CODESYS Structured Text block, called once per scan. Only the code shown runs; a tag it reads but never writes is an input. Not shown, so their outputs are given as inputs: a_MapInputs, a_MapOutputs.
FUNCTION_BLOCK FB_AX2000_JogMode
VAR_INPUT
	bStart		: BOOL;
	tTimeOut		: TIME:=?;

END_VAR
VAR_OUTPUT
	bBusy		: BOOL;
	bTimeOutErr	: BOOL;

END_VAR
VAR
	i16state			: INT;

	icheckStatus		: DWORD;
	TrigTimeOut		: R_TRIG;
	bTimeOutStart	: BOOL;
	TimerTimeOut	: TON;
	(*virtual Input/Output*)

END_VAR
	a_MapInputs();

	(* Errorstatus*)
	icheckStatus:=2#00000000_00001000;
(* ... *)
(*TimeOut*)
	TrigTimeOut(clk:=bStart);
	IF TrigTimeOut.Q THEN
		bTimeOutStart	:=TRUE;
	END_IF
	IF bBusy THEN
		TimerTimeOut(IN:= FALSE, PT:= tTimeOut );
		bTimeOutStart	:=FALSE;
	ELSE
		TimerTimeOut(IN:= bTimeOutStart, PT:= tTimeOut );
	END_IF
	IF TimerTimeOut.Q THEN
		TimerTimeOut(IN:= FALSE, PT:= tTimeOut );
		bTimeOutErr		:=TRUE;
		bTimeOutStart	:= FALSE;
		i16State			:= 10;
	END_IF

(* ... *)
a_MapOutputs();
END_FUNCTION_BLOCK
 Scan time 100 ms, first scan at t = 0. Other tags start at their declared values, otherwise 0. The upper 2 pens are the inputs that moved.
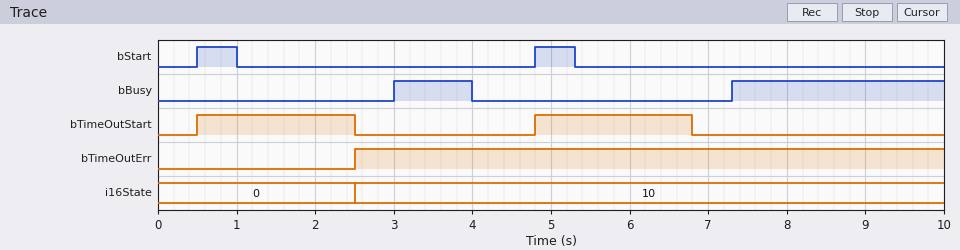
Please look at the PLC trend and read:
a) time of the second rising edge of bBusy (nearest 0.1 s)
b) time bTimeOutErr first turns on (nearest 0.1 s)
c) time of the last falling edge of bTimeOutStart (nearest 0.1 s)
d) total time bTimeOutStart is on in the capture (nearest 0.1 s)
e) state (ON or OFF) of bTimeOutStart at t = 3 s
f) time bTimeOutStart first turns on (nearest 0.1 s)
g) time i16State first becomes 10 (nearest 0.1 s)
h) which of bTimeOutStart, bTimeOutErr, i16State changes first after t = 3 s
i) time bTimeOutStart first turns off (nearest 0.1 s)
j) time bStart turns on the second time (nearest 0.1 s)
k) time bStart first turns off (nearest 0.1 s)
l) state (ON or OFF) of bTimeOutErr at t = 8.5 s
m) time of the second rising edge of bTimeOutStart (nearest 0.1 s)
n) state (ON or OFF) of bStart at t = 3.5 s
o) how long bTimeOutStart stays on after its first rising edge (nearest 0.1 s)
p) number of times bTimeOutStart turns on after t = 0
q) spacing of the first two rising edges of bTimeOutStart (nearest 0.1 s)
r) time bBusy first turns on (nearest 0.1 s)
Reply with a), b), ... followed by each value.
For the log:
a) 7.3 s
b) 2.5 s
c) 6.8 s
d) 4.0 s
e) OFF
f) 0.5 s
g) 2.5 s
h) bTimeOutStart
i) 2.5 s
j) 4.8 s
k) 1.0 s
l) ON
m) 4.8 s
n) OFF
o) 2.0 s
p) 2
q) 4.3 s
r) 3.0 s
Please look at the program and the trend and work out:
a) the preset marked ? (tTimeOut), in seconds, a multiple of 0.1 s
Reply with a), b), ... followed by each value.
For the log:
a) 2.0 s
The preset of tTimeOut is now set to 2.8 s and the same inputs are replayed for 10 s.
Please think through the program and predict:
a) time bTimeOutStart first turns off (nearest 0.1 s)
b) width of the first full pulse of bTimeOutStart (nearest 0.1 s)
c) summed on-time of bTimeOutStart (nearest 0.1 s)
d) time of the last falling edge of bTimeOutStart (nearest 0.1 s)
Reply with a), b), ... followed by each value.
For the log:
a) 3.0 s
b) 2.5 s
c) 5.0 s
d) 7.3 s
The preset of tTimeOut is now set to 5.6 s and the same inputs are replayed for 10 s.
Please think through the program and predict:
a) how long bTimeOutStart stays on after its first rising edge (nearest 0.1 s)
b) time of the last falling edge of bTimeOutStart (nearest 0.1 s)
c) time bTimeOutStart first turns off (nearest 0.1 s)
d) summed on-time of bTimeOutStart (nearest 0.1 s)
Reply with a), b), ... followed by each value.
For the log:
a) 2.5 s
b) 7.3 s
c) 3.0 s
d) 5.0 s
